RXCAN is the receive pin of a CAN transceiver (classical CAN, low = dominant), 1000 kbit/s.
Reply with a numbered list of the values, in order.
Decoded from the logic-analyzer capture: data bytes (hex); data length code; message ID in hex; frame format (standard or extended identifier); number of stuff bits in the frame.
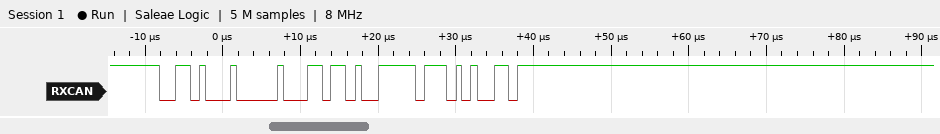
1. B4
2. 1
3. 0x344
4. standard
5. 2
